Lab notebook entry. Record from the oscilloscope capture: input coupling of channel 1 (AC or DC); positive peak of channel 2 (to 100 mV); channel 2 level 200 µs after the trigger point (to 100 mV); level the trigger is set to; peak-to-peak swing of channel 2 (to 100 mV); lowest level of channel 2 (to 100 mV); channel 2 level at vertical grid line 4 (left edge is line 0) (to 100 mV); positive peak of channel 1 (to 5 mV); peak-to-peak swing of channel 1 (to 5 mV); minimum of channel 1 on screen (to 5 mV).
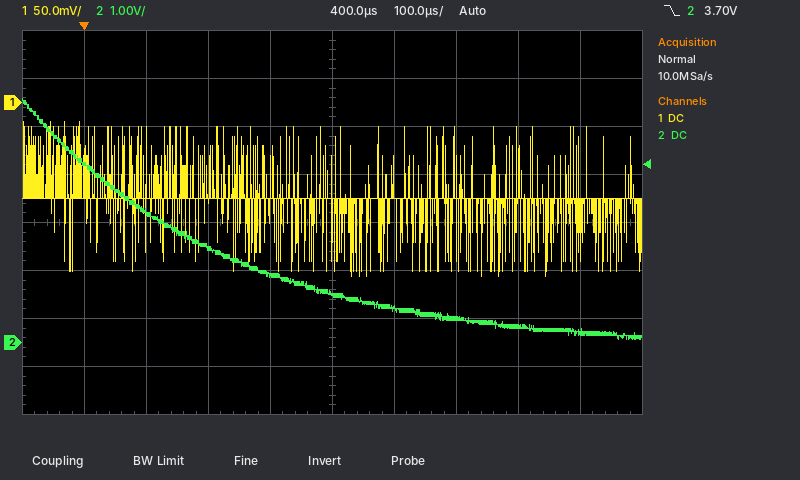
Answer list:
DC
5.1 V
2.0 V
3.70 V
5.0 V
100 mV
1.4 V
-20 mV
160 mV
-180 mV
